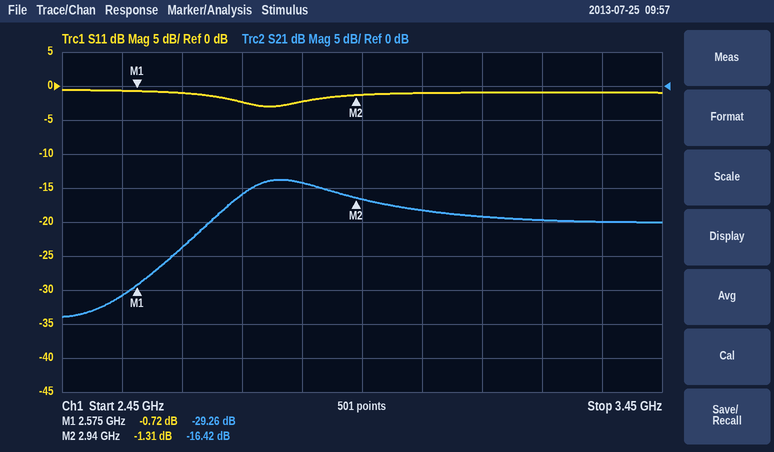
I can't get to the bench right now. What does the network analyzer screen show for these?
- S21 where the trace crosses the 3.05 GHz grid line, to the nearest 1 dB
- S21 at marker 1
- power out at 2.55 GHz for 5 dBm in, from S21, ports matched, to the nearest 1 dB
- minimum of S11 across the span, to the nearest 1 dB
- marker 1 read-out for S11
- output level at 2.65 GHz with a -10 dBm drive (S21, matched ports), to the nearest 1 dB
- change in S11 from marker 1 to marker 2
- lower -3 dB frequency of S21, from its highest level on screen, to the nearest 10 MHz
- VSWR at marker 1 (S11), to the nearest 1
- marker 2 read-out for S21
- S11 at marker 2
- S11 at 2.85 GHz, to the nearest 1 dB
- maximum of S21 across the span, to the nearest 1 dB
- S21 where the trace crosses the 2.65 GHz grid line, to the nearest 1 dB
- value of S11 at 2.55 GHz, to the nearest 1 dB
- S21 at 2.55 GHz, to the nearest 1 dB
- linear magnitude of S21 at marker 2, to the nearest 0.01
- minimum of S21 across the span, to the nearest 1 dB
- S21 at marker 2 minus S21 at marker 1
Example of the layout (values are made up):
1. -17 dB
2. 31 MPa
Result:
1. -18 dB
2. -29.26 dB
3. -26 dBm
4. -3 dB
5. -0.72 dB
6. -34 dBm
7. -0.59 dB
8. 2.74 GHz
9. 24
10. -16.42 dB
11. -1.31 dB
12. -2 dB
13. -14 dB
14. -24 dB
15. -1 dB
16. -31 dB
17. 0.15
18. -34 dB
19. 12.84 dB
